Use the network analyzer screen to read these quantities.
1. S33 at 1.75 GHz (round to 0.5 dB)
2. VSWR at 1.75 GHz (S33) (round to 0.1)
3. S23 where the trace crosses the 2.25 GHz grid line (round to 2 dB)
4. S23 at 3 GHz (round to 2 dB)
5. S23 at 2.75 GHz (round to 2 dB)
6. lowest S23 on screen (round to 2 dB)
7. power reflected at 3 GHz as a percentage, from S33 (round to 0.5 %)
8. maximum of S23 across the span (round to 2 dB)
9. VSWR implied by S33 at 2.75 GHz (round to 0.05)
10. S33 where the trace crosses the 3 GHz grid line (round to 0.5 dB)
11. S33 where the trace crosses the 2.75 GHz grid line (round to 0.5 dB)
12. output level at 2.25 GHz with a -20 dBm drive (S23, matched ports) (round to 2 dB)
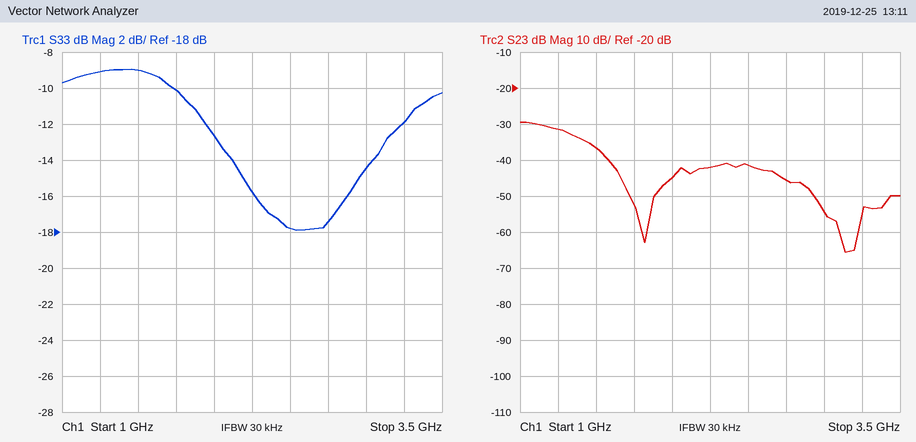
-10.0 dB
1.9
-42 dB
-54 dB
-46 dB
-66 dB
3.5 %
-30 dB
1.30
-14.5 dB
-17.5 dB
-62 dBm
